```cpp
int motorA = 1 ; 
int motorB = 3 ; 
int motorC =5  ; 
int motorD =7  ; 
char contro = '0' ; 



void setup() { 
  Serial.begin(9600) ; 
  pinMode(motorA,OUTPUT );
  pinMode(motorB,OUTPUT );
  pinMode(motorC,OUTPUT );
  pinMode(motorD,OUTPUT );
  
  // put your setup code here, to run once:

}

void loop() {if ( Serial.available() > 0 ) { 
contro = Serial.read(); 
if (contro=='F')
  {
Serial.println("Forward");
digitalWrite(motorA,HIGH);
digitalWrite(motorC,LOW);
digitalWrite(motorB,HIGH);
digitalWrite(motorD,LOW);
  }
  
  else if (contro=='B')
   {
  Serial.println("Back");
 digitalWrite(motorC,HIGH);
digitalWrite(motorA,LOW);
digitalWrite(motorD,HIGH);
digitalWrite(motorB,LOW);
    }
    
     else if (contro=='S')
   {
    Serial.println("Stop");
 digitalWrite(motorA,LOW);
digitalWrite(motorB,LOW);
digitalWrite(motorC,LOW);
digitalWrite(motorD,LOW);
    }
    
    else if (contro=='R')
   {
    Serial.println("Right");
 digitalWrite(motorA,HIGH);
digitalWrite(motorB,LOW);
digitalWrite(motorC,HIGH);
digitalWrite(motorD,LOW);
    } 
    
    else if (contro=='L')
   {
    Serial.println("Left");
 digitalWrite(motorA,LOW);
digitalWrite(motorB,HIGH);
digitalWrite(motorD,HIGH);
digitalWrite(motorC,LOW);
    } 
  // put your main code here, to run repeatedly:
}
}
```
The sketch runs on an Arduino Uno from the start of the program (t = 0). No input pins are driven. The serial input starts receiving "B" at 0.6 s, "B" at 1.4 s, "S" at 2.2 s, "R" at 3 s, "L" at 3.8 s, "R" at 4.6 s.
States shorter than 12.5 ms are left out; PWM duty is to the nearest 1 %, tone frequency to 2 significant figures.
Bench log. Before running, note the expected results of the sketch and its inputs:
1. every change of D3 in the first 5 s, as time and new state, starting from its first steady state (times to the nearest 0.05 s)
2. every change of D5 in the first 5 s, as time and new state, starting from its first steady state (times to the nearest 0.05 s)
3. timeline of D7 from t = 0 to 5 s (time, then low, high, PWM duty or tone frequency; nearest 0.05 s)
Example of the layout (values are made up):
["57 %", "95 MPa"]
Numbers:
["0 s low; 3.8 s high; 4.6 s low", "0 s low; 0.6 s high; 2.2 s low; 3 s high; 3.8 s low; 4.6 s high", "0 s low; 0.6 s high; 2.2 s low; 3.8 s high; 4.6 s low"]
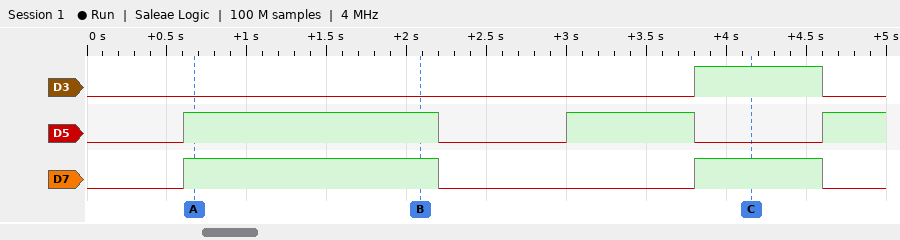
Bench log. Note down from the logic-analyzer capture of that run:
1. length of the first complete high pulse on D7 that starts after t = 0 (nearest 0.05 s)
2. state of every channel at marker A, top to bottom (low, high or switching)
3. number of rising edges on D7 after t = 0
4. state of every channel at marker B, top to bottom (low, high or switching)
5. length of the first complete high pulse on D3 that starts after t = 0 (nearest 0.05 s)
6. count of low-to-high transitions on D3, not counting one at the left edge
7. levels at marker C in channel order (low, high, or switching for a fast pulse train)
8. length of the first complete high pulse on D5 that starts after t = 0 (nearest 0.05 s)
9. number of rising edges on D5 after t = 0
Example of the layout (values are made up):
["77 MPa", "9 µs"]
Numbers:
["1.60 s", "D3 low, D5 high, D7 high", "2", "D3 low, D5 high, D7 high", "0.80 s", "1", "D3 high, D5 low, D7 high", "1.60 s", "3"]
